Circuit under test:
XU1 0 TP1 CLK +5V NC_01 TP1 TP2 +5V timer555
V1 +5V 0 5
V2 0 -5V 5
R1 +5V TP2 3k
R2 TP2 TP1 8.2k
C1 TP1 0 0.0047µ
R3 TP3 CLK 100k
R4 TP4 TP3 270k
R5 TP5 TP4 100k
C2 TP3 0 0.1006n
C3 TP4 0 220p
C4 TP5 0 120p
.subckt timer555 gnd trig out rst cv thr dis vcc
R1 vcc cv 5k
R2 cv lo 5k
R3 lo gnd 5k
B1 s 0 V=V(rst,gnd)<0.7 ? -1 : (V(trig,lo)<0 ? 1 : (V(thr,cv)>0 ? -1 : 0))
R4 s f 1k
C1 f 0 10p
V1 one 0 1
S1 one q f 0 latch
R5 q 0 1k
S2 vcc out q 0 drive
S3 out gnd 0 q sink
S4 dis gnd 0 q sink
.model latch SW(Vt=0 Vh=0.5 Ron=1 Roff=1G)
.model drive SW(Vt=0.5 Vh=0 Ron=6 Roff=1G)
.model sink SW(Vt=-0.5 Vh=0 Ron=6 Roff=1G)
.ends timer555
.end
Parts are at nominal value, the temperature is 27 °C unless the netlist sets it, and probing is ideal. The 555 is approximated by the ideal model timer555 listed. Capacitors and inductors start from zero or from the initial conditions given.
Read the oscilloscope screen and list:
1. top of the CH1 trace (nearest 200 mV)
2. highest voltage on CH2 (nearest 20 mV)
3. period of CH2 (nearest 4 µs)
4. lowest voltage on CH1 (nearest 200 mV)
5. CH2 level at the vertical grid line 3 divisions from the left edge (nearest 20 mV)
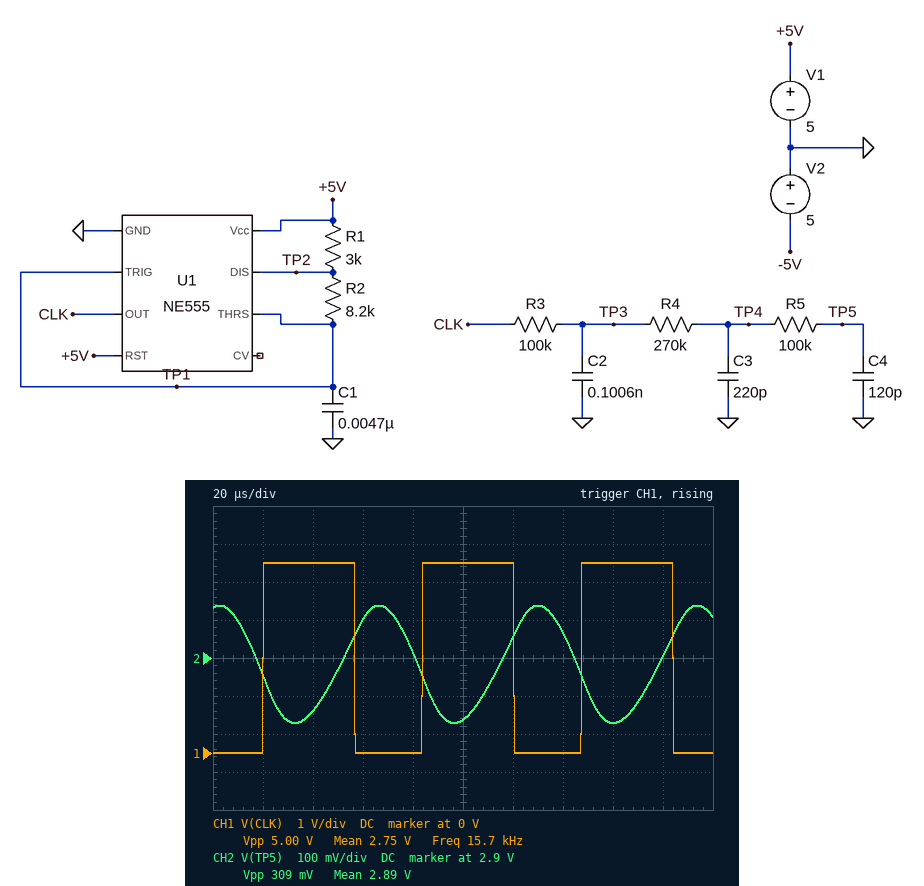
5.0 V
3.04 V
64 µs
0 V
3.00 V
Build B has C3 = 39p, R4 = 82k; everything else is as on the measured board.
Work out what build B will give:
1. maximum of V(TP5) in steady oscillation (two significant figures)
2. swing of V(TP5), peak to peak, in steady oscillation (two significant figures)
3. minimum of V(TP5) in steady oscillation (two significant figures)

3.5 V
1.3 V
2.2 V
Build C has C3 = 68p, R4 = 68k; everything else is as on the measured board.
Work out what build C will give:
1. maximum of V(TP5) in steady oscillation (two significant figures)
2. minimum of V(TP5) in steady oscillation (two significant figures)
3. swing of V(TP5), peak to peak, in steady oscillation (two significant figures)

3.5 V
2.3 V
1.2 V
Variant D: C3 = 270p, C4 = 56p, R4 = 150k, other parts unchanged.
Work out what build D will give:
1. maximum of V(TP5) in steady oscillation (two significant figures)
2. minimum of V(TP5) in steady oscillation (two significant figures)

3.2 V
2.6 V
